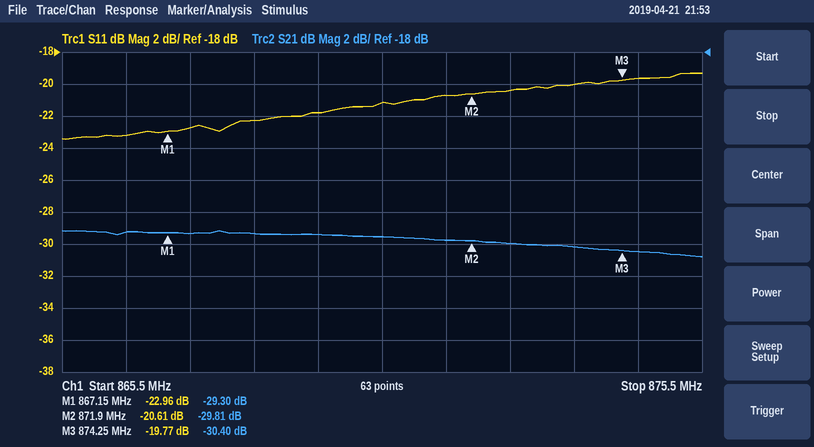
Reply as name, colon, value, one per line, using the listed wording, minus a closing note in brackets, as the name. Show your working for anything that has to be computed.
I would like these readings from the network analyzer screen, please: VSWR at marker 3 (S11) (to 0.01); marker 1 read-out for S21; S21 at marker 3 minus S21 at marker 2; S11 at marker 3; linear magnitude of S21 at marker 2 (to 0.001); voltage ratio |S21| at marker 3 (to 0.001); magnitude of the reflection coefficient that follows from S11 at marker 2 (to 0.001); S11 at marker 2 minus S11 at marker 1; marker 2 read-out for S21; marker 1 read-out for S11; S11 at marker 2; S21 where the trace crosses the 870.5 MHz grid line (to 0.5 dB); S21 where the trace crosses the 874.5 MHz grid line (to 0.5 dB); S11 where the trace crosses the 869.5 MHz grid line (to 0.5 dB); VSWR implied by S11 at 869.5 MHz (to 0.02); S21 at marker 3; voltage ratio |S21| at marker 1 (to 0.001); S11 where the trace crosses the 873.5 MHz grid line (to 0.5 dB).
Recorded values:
VSWR at marker 3 (S11): (1 + 0.1027)/(1 − 0.1027) ≈ 1.23
marker 1 read-out for S21: -29.30 dB
S21 at marker 3 minus S21 at marker 2: -30.4 − (-29.81) = -0.59 dB
S11 at marker 3: -19.77 dB
linear magnitude of S21 at marker 2: 10^(-29.81/20) ≈ 0.032
voltage ratio |S21| at marker 3: 10^(-30.4/20) ≈ 0.030
magnitude of the reflection coefficient that follows from S11 at marker 2: 10^(-20.61/20) ≈ 0.093
S11 at marker 2 minus S11 at marker 1: -20.61 − (-22.96) = 2.35 dB
marker 2 read-out for S21: -29.81 dB
marker 1 read-out for S11: -22.96 dB
S11 at marker 2: -20.61 dB
S21 where the trace crosses the 870.5 MHz grid line: -29.5 dB
S21 where the trace crosses the 874.5 MHz grid line: -30.5 dB
S11 where the trace crosses the 869.5 MHz grid line: -22.0 dB
VSWR implied by S11 at 869.5 MHz: |Γ| = 10^(-22/20) = 0.0794; VSWR = (1 + 0.0794)/(1 − 0.0794) ≈ 1.17, so 1.18 to the nearest 0.02
S21 at marker 3: -30.40 dB
voltage ratio |S21| at marker 1: 10^(-29.3/20) ≈ 0.034
S11 where the trace crosses the 873.5 MHz grid line: -20.0 dB
